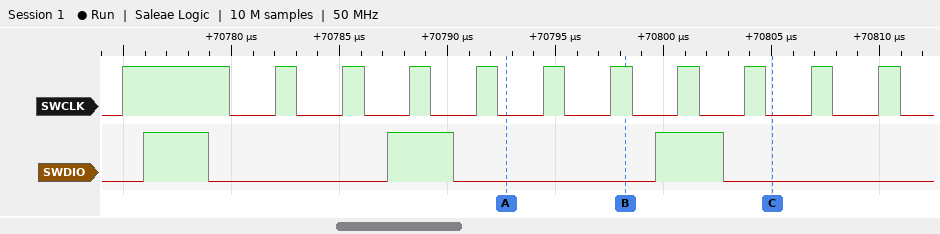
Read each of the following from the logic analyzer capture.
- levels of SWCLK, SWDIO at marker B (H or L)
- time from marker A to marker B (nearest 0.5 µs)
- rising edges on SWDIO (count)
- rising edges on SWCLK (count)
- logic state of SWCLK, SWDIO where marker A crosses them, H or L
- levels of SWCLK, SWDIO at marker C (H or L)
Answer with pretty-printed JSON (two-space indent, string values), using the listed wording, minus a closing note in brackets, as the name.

{
  "levels of SWCLK, SWDIO at marker B": "SWCLK=H, SWDIO=L",
  "time from marker A to marker B": "5.5 µs",
  "rising edges on SWDIO": "3",
  "rising edges on SWCLK": "11",
  "logic state of SWCLK, SWDIO where marker A crosses them, H or L": "SWCLK=L, SWDIO=L",
  "levels of SWCLK, SWDIO at marker C": "SWCLK=L, SWDIO=L"
}
